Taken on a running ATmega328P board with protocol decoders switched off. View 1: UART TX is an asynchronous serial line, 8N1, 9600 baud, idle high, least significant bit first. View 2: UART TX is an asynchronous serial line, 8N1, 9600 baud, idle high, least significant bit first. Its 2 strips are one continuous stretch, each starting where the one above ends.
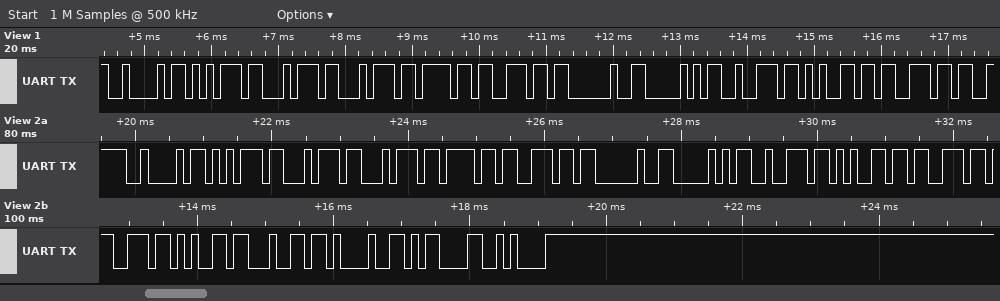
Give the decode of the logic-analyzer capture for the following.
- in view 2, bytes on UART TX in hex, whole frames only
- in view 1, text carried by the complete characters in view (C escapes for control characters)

0x42 0x75 0x74 0x74 0x6F 0x6E 0x20 0x50 0x72 0x65 0x73 0x73 0x65 0x64 0x21 0x0D 0x0A
"Button Pres"
